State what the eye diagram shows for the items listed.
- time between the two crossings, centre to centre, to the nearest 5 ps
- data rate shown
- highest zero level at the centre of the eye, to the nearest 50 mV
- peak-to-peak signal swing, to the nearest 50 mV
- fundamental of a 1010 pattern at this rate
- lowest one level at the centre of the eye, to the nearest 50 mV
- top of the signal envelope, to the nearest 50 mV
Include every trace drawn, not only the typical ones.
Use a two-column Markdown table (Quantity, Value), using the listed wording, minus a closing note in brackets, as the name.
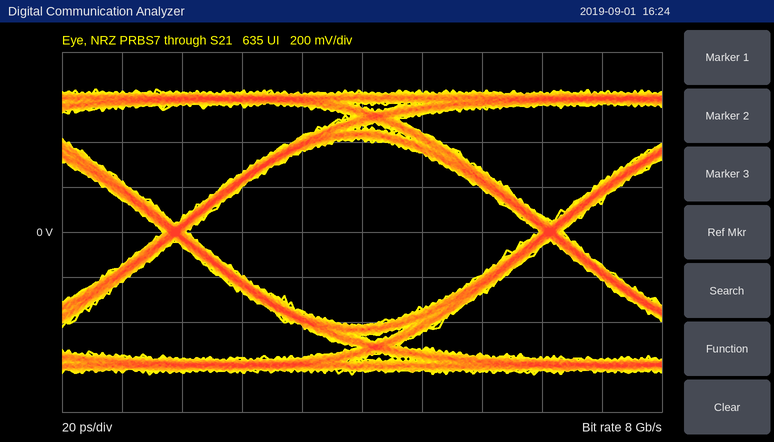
| Quantity | Value |
|---|---|
| time between the two crossings, centre to centre, to the nearest 5 ps | 125 ps |
| data rate shown | 8 Gb/s |
| highest zero level at the centre of the eye, to the nearest 50 mV | -400 mV |
| peak-to-peak signal swing, to the nearest 50 mV | 1.25 V |
| fundamental of a 1010 pattern at this rate | 4 GHz |
| lowest one level at the centre of the eye, to the nearest 50 mV | 400 mV |
| top of the signal envelope, to the nearest 50 mV | 650 mV |
